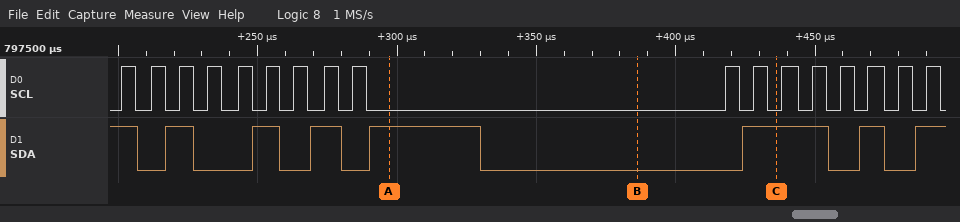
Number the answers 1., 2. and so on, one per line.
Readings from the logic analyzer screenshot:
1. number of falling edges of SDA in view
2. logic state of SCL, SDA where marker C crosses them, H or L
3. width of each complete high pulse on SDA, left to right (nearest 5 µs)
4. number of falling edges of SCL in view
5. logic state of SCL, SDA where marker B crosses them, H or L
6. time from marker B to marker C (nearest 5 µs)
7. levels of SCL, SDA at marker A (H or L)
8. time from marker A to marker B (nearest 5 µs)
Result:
1. 7
2. SCL=L, SDA=H
3. 10 µs, 10 µs, 10 µs, 40 µs, 30 µs, 10 µs
4. 17
5. SCL=L, SDA=L
6. 50 µs
7. SCL=L, SDA=H
8. 90 µs
